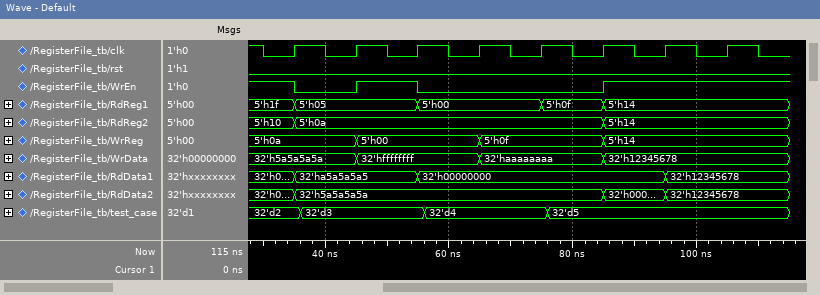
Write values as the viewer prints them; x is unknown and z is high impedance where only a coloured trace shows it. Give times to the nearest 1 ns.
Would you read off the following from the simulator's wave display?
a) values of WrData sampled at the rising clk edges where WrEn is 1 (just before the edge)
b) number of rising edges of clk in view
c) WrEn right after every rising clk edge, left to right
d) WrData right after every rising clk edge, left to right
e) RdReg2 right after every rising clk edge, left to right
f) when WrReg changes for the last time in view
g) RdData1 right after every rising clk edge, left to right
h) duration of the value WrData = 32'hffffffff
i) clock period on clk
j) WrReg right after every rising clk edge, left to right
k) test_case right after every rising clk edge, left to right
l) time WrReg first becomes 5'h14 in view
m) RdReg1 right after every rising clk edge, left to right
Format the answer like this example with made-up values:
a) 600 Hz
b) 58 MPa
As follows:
a) 32'h5a5a5a5a, 32'hffffffff, 32'h12345678, 32'h12345678
b) 8
c) 0 1 0 0 0 1 1 1
d) 32'h5a5a5a5a, 32'hffffffff, 32'hffffffff, 32'haaaaaaaa, 32'haaaaaaaa, 32'h12345678, 32'h12345678, 32'h12345678
e) 5'h0a, 5'h0a, 5'h0a, 5'h0a, 5'h0a, 5'h14, 5'h14, 5'h14
f) 85 ns
g) 32'ha5a5a5a5, 32'ha5a5a5a5, 32'h00000000, 32'h00000000, 32'h00000000, 32'h00000000, 32'h12345678, 32'h12345678
h) 20 ns
i) 10 ns
j) 5'h0a, 5'h00, 5'h00, 5'h0f, 5'h0f, 5'h14, 5'h14, 5'h14
k) 32'd2, 32'd3, 32'd3, 32'd4, 32'd4, 32'd5, 32'd5, 32'd5
l) 85 ns
m) 5'h05, 5'h05, 5'h00, 5'h00, 5'h0f, 5'h14, 5'h14, 5'h14
